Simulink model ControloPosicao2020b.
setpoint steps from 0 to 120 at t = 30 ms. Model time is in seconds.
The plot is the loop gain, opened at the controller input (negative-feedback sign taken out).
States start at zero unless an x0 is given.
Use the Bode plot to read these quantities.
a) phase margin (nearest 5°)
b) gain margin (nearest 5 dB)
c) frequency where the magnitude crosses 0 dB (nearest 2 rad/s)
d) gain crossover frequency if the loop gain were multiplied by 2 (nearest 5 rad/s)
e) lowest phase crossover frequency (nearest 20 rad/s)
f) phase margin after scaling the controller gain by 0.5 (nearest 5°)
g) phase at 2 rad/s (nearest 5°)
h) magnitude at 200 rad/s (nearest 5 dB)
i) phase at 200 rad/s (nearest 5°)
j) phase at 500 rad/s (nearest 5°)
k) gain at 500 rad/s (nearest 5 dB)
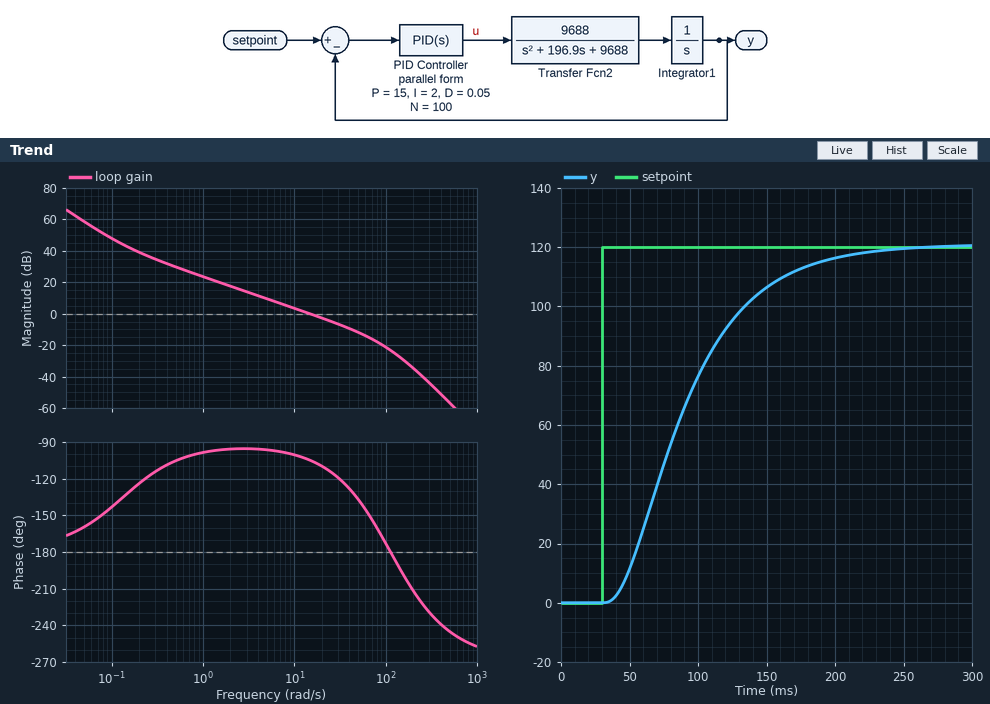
75°
25 dB
14 rad/s
30 rad/s
120 rad/s
80°
-95°
-35 dB
-210°
-245°
-55 dB
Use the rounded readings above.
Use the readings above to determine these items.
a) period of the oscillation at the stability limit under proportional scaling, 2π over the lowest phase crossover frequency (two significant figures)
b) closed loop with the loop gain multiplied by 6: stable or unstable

0.052 s
stable
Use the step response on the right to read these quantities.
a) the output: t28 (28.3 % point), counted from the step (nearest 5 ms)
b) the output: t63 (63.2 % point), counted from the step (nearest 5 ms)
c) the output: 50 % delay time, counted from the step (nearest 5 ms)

35 ms
70 ms
55 ms
